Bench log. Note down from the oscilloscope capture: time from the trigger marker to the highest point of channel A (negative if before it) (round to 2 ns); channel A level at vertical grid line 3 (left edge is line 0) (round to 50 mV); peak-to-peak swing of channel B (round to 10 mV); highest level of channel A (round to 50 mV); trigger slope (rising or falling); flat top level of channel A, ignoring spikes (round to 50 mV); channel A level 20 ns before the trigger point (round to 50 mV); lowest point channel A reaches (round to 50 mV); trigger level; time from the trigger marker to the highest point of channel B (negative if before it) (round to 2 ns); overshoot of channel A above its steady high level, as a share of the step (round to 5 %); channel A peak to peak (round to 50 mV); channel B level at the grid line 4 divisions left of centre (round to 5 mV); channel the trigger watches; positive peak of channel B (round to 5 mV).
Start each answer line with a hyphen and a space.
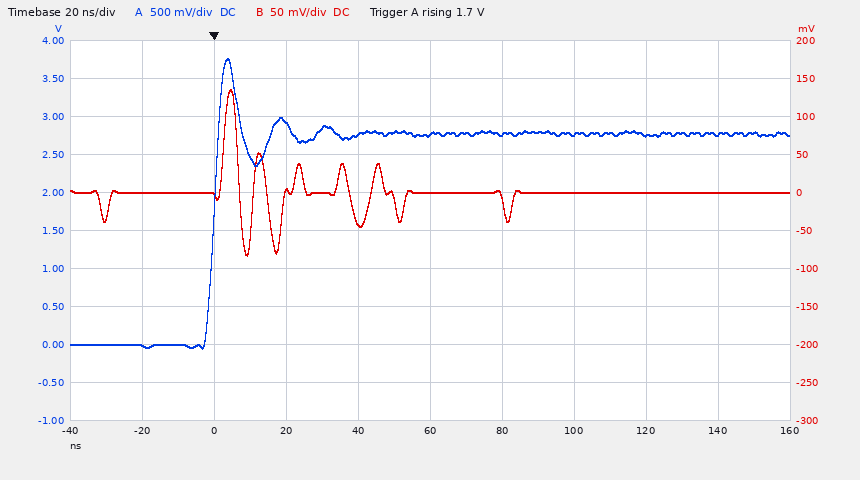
- +4 ns
- 2.90 V
- 220 mV
- 3.75 V
- rising
- 2.80 V
- 0 mV
- -50 mV
- 1.7 V
- +4 ns
- 35 %
- 3.80 V
- 0 mV
- channel A
- 135 mV
